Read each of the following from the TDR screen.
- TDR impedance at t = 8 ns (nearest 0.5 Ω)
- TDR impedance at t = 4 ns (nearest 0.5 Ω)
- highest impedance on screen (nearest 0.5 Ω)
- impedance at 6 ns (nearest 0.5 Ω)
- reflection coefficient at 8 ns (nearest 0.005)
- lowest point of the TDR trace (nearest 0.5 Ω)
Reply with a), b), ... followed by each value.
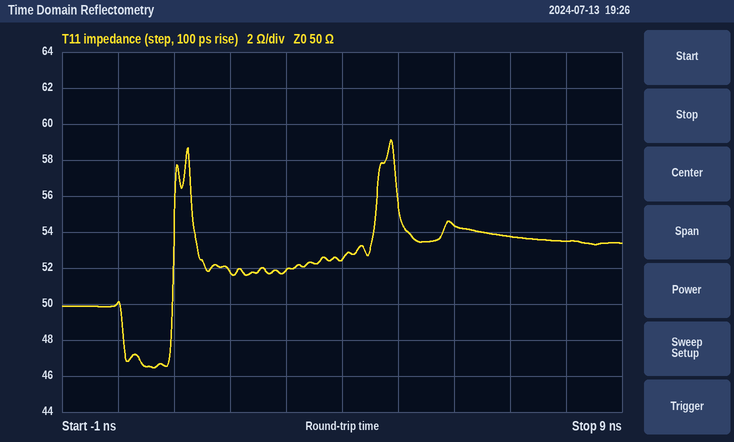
a) 53.5 Ω
b) 52.5 Ω
c) 59.0 Ω
d) 54.5 Ω
e) +0.035
f) 46.5 Ω
